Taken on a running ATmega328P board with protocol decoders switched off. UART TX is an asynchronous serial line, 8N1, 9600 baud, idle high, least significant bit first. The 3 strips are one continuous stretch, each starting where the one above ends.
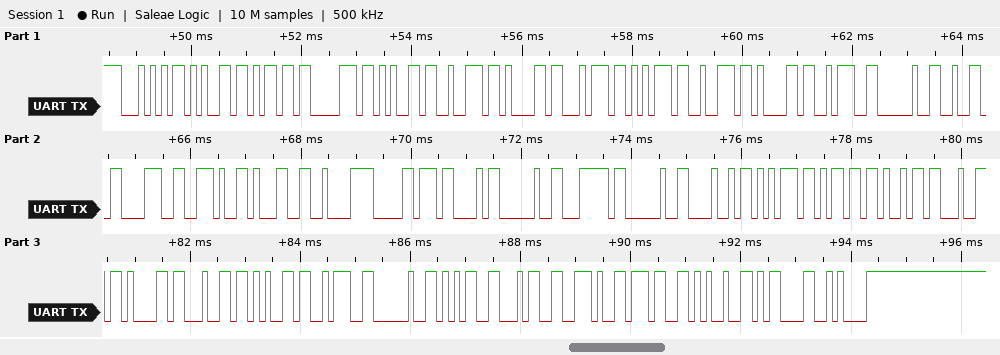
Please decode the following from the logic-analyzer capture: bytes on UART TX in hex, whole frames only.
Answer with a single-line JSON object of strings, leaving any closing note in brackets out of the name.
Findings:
{"bytes on UART TX in hex, whole frames only": "54 65 6D 70 65 72 61 74 75 72 61 3A 20 32 38 2E 31 C2 B0 43 20 7C 20 48 75 6D 69 64 61 64 65 3A 20 35 34 2E 37 25 0D 0A"}
